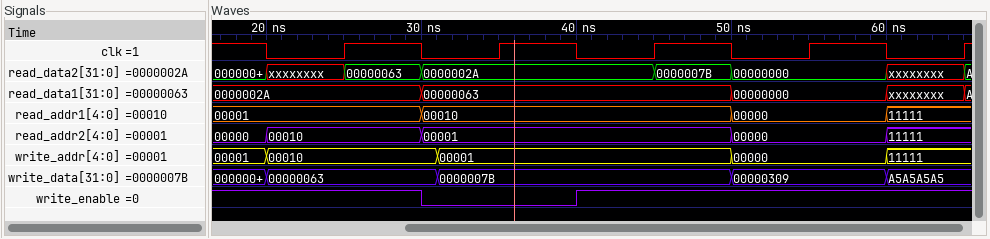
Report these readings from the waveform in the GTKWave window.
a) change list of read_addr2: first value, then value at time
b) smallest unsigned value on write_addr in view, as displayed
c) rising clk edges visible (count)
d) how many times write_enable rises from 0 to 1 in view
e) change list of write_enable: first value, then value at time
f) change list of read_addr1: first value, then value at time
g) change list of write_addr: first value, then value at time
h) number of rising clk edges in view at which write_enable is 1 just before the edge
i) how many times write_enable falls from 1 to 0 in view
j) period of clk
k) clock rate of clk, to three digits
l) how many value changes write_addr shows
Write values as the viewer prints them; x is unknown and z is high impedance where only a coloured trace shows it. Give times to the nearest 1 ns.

00000, 00010 at 20 ns, 00001 at 30 ns, 00000 at 50 ns, 11111 at 60 ns
00000
5
1
1, 0 at 30 ns, 1 at 40 ns
00001, 00010 at 30 ns, 00000 at 50 ns, 11111 at 60 ns
00001, 00010 at 20 ns, 00001 at 31 ns, 00000 at 50 ns, 11111 at 60 ns
4
1
10 ns
100 MHz
4
